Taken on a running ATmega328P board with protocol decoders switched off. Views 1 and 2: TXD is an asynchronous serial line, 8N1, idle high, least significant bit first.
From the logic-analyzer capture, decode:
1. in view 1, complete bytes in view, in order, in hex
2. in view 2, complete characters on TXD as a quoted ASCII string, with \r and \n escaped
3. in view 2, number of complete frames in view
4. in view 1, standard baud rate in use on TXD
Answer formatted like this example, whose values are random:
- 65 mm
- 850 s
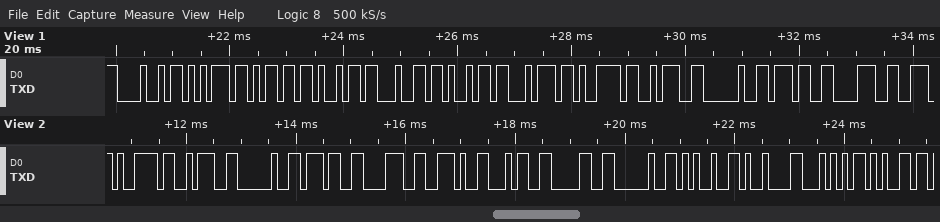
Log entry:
- 48 75 6D 69 64 69 74 79 3A 20 37 38
- "y: 78.40 %\tTe"
- 13
- 9600 baud
